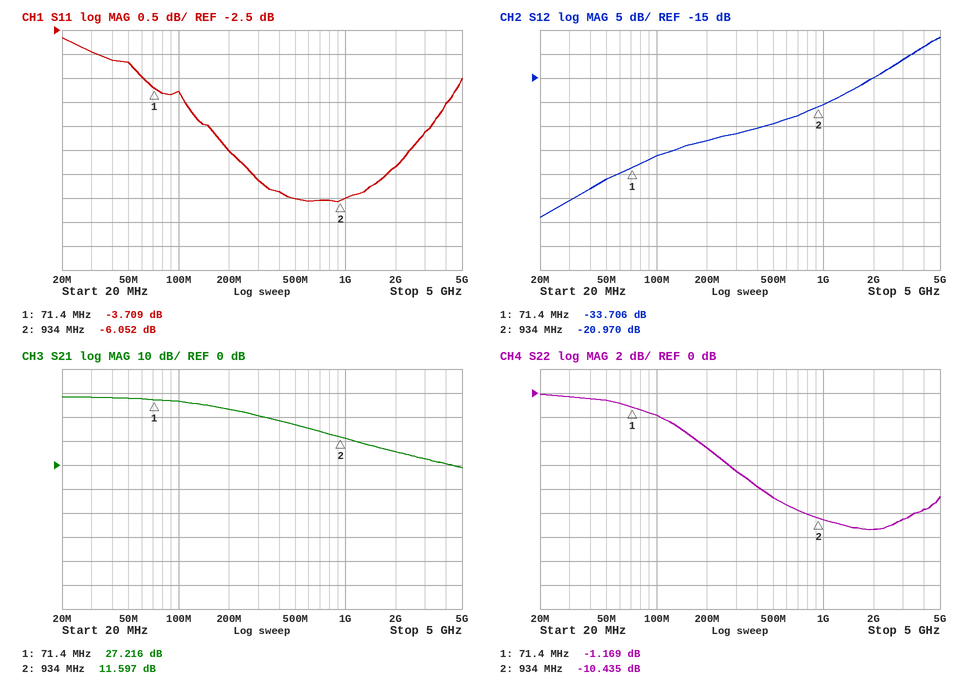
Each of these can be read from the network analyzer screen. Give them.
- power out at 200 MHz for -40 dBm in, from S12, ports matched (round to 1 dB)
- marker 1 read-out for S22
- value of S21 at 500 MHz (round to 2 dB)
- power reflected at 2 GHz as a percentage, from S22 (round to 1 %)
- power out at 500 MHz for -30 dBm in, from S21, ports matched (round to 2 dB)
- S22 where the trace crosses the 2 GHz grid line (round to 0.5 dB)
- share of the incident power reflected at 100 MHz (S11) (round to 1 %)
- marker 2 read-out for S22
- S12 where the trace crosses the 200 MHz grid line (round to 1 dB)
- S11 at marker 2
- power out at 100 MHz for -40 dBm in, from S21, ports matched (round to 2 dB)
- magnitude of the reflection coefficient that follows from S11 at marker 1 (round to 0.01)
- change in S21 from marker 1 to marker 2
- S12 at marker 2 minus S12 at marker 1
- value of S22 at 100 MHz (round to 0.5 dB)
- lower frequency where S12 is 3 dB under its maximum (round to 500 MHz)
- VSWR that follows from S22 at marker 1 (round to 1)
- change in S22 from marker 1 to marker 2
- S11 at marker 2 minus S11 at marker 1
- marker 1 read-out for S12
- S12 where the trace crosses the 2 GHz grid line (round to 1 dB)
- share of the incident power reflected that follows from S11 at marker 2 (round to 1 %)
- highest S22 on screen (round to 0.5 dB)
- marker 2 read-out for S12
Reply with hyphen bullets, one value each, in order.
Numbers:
- -68 dBm
- -1.169 dB
- 16 dB
- 7 %
- -14 dBm
- -11.5 dB
- 42 %
- -10.435 dB
- -28 dB
- -6.052 dB
- -14 dBm
- 0.65
- -15.619 dB
- 12.736 dB
- -2.0 dB
- 3.5 GHz
- 15
- -9.266 dB
- -2.343 dB
- -33.706 dB
- -15 dB
- 25 %
- 0.0 dB
- -20.970 dB
